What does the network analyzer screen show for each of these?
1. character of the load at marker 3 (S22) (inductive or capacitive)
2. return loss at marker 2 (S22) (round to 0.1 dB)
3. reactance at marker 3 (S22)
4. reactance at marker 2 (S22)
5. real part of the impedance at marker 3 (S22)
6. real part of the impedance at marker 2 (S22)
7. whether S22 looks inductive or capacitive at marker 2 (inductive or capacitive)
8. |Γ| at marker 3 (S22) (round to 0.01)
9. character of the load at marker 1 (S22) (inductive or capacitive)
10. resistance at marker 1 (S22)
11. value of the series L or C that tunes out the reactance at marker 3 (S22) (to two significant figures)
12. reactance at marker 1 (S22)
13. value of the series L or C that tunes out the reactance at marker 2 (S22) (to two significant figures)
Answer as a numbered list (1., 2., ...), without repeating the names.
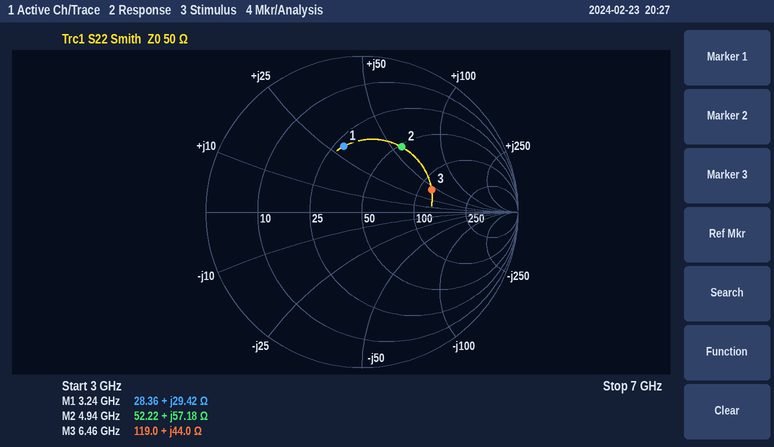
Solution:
1. inductive
2. 6.2 dB
3. +44.0 Ω
4. +57.18 Ω
5. 119.0 Ω
6. 52.22 Ω
7. inductive
8. 0.47
9. inductive
10. 28.36 Ω
11. 560 fF
12. +29.42 Ω
13. 560 fF
